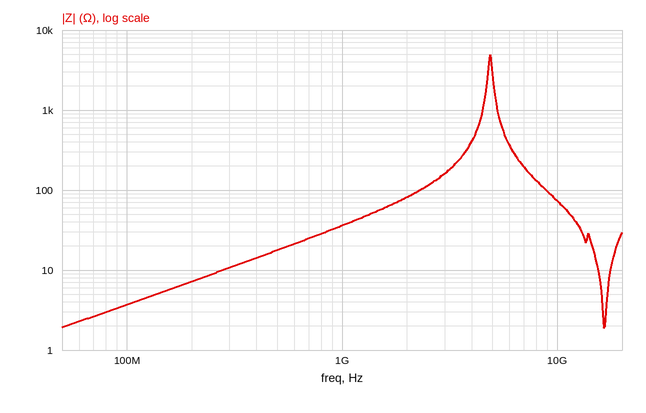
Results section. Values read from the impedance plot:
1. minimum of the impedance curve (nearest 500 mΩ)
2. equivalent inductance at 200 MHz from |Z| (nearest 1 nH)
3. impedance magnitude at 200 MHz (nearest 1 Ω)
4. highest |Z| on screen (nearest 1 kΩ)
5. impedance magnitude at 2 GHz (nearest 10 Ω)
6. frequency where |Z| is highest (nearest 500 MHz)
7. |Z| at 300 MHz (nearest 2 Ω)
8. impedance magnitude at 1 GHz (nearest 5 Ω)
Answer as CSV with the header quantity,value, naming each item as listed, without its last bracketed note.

quantity,value
minimum of the impedance curve,2.0 Ω
equivalent inductance at 200 MHz from |Z|,6 nH
impedance magnitude at 200 MHz,7 Ω
highest |Z| on screen,5 kΩ
impedance magnitude at 2 GHz,80 Ω
frequency where |Z| is highest,5.0 GHz
|Z| at 300 MHz,10 Ω
impedance magnitude at 1 GHz,35 Ω
